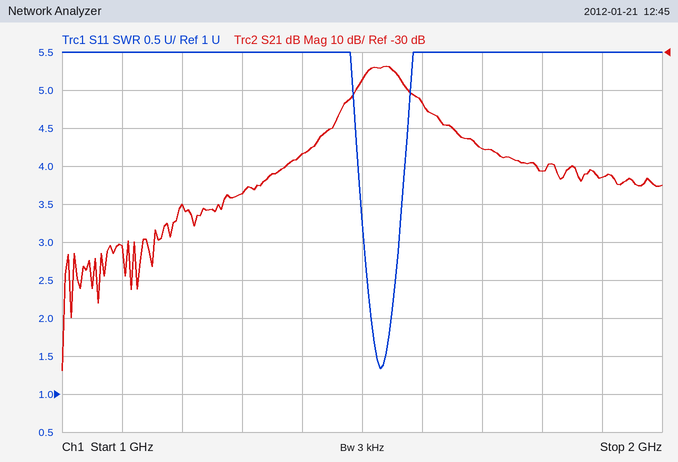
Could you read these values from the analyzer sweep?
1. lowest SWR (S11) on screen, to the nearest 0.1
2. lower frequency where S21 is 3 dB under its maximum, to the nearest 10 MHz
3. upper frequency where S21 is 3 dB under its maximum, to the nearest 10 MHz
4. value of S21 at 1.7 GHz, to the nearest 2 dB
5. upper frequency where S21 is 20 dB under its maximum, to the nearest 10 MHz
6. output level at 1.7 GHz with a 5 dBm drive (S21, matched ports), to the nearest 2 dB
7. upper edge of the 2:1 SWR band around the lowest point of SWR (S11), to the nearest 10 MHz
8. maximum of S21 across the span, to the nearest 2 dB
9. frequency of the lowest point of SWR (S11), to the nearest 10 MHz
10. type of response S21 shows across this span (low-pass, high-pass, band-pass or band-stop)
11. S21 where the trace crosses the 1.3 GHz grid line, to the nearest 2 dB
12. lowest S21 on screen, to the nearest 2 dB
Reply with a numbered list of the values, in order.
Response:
1. 1.3
2. 1.50 GHz
3. 1.56 GHz
4. -56 dB
5. 1.69 GHz
6. -50 dBm
7. 1.55 GHz
8. -34 dB
9. 1.53 GHz
10. band-pass
11. -68 dB
12. -114 dB
